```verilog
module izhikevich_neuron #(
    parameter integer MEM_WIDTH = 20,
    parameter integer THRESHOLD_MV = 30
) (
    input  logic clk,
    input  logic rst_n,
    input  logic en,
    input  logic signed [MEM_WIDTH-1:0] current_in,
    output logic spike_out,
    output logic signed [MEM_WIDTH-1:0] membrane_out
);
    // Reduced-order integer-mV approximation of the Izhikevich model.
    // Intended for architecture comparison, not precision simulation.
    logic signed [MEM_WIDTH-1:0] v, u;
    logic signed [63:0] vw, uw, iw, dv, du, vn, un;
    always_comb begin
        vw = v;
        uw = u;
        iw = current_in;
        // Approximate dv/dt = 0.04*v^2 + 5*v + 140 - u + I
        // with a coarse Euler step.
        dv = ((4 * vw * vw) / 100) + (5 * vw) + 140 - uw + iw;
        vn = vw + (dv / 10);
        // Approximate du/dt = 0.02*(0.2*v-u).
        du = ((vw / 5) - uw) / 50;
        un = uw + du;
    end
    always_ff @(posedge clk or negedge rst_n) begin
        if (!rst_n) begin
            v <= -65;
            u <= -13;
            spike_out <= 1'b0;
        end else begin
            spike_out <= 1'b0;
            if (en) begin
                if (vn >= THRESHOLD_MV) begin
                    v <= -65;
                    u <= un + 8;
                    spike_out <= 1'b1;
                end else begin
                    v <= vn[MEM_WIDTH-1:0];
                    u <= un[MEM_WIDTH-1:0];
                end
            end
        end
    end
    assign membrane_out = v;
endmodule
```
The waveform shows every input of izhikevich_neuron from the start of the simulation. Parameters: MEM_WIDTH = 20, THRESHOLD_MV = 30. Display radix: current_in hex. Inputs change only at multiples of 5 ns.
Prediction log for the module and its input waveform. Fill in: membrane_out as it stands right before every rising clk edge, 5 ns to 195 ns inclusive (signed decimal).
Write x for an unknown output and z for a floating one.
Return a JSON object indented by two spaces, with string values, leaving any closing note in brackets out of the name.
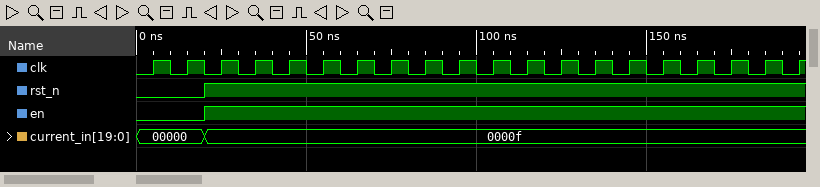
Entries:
{
  "membrane_out as it stands right before every rising clk edge, 5 ns to 195 ns inclusive": "-65, -65, -65, -64, -63, -62, -61, -60, -59, -58, -57, -56, -55, -54, -53, -52, -51, -50, -49, -48"
}
